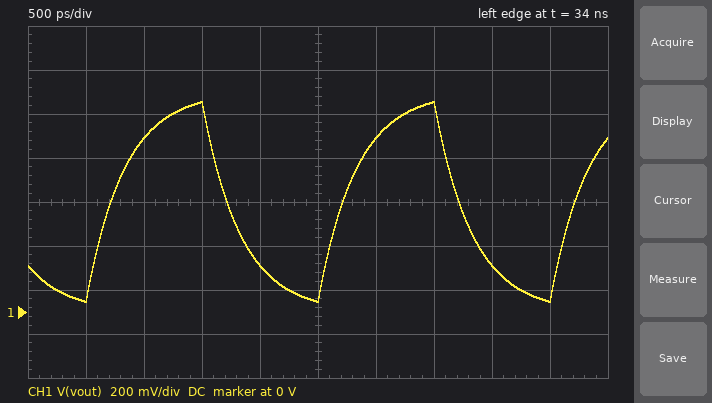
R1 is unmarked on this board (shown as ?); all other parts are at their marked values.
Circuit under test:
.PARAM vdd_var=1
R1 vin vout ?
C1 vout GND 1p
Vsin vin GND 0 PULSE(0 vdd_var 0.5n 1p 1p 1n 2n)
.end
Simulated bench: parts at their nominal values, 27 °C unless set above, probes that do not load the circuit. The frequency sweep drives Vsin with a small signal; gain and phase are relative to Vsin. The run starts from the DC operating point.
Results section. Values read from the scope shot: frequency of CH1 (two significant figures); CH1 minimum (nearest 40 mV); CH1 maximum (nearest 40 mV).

500 MHz
40 mV
960 mV
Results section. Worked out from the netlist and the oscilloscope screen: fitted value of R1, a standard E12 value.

330 Ω
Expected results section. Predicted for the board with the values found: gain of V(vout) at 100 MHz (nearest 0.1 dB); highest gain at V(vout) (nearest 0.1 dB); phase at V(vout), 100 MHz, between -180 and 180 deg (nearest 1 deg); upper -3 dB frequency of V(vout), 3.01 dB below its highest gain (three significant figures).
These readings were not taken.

-0.2 dB
0 dB
-12 deg
482 MHz
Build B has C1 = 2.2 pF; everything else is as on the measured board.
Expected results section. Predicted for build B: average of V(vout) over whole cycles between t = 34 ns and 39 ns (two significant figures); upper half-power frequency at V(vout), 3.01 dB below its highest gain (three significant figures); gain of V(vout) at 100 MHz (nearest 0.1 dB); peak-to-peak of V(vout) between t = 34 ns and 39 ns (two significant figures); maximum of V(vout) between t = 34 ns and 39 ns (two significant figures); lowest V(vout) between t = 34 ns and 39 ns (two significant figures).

500 mV
219 MHz
-0.8 dB
600 mV
800 mV
200 mV
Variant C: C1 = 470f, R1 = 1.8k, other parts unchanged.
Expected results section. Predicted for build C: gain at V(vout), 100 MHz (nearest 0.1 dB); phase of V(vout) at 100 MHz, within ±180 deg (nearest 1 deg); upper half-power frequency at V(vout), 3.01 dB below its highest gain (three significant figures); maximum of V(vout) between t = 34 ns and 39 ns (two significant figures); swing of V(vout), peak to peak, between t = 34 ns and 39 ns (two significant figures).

-1.1 dB
-28 deg
188 MHz
770 mV
530 mV
